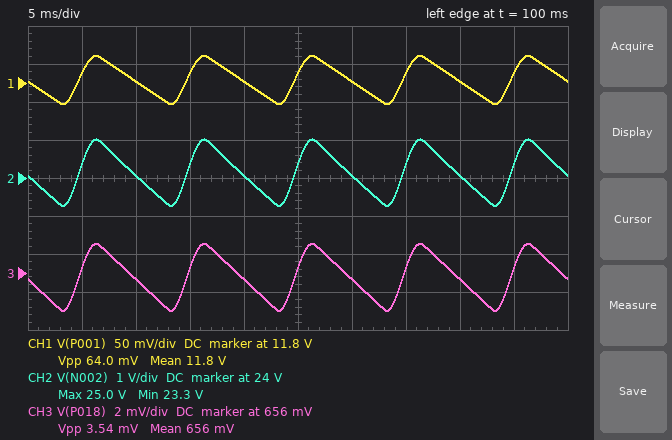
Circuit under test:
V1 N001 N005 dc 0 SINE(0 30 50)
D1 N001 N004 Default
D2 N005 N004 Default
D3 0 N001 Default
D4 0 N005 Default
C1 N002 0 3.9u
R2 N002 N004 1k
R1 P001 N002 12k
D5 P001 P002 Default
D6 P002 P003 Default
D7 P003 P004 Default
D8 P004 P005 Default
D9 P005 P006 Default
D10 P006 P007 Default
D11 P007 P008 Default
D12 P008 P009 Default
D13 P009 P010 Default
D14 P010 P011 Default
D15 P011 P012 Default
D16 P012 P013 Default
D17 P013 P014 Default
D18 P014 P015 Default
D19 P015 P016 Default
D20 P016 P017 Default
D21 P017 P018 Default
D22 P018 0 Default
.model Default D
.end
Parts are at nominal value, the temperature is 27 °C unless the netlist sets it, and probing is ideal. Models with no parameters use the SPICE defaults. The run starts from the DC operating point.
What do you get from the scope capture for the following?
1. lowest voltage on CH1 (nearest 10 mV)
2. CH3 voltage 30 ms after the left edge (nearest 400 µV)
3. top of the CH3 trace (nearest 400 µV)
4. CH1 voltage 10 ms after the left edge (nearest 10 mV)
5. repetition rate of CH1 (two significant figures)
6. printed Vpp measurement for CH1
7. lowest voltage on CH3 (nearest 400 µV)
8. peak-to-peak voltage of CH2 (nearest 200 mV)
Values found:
11.77 V
655.6 mV
657.6 mV
11.80 V
100 Hz
64.0 mV
654.0 mV
1.8 V
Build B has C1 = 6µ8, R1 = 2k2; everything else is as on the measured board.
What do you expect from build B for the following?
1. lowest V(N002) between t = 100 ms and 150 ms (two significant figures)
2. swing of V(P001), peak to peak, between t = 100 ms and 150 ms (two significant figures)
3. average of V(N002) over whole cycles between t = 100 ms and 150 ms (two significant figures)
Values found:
18 V
150 mV
19 V
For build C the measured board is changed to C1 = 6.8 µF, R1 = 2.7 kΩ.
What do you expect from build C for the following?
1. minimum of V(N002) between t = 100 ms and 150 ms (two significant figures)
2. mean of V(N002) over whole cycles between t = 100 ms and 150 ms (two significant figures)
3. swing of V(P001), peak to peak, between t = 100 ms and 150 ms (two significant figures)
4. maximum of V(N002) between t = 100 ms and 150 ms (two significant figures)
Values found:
19 V
20 V
130 mV
21 V
